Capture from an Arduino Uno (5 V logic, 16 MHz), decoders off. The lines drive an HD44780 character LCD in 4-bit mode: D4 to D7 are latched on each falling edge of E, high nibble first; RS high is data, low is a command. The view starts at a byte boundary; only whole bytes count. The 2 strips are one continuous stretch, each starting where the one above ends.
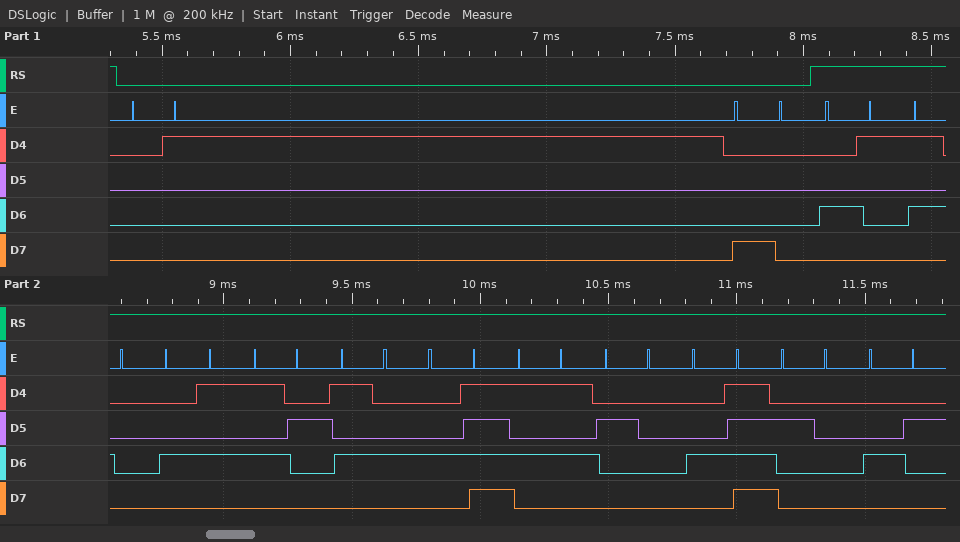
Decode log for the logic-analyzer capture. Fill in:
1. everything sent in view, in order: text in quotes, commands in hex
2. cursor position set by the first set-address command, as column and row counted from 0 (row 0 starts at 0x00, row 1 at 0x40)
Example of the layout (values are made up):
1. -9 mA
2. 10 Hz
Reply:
1. 0x01 0x80 "APERTOU O B"
2. column 0, row 0
